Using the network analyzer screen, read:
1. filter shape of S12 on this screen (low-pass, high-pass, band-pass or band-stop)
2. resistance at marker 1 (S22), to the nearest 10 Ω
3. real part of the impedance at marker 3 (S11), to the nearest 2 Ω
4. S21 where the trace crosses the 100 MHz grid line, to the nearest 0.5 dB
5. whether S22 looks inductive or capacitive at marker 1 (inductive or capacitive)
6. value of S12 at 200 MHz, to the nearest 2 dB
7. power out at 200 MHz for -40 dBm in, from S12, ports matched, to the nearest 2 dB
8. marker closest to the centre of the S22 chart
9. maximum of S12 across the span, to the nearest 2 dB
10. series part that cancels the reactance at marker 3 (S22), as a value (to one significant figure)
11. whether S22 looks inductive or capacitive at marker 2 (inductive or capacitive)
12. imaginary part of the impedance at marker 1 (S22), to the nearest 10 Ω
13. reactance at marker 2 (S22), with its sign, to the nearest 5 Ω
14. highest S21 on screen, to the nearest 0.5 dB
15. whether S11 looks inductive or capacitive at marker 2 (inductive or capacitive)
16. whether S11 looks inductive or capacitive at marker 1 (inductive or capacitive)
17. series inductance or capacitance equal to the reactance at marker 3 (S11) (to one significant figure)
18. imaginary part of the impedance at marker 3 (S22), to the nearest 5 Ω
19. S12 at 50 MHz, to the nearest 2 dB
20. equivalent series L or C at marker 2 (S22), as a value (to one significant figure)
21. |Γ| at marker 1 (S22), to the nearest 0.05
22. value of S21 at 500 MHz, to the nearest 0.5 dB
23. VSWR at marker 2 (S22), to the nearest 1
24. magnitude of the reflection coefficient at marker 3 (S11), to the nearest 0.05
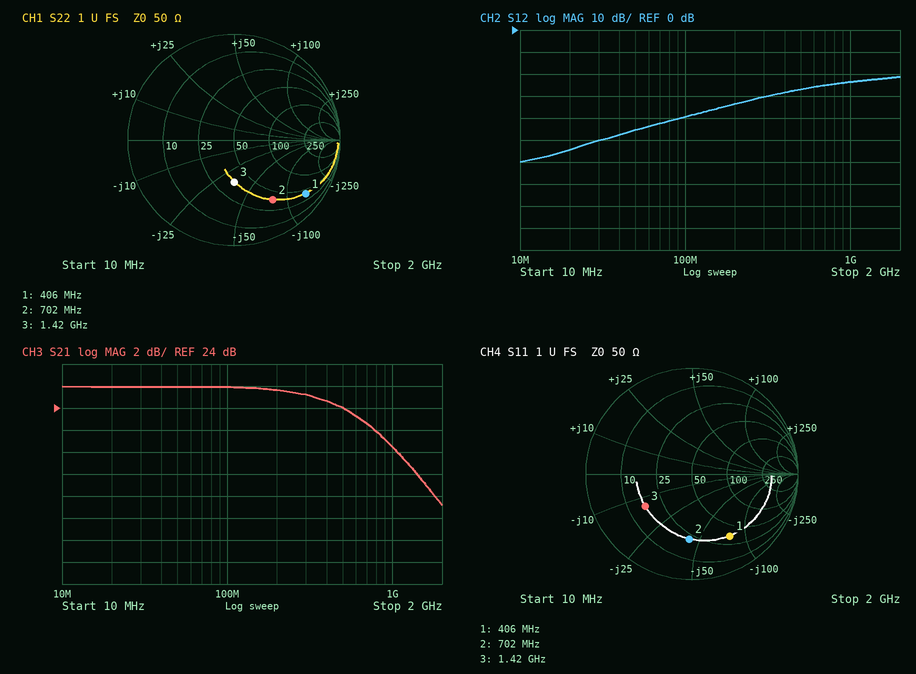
high-pass
40 Ω
16 Ω
26.0 dB
capacitive
-34 dB
-74 dBm
marker 3
-22 dB
4 nH
capacitive
-140 Ω
-80 Ω
26.0 dB
capacitive
capacitive
8 pF
-35 Ω
-46 dB
3 pF
0.85
24.0 dB
5
0.55
